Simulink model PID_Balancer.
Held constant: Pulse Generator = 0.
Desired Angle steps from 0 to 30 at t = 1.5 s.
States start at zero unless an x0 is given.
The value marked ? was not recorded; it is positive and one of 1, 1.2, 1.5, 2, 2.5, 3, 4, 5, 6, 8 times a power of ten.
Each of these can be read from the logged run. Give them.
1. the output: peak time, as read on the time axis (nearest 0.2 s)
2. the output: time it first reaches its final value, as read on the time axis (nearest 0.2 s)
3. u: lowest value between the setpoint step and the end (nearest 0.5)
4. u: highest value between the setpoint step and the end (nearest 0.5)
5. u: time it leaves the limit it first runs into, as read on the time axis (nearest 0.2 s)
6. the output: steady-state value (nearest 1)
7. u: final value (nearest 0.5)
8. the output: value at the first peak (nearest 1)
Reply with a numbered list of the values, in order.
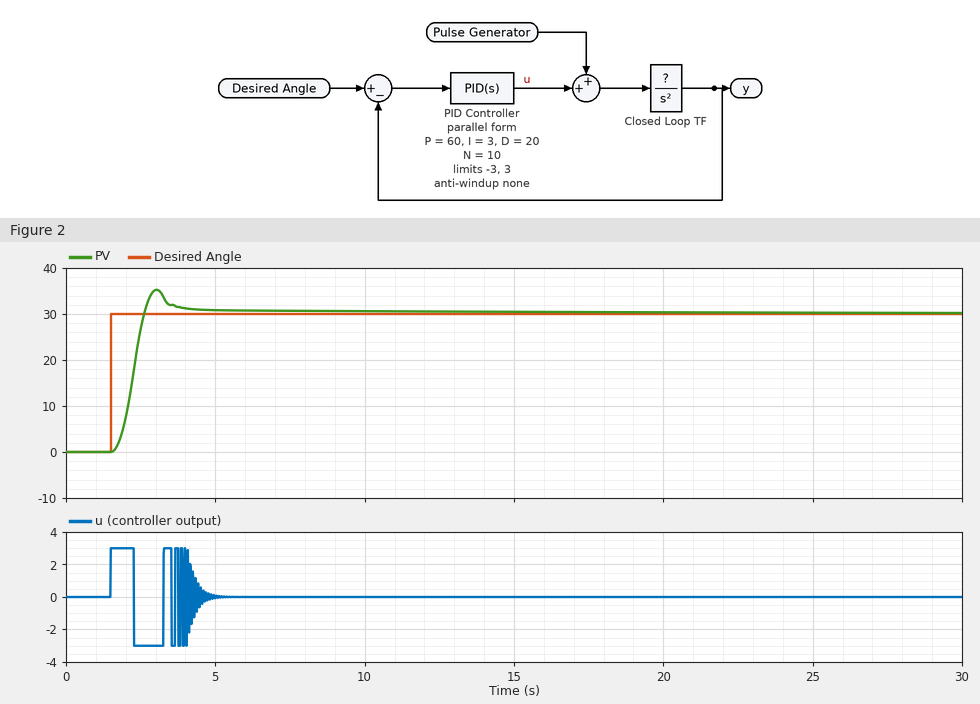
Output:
1. 3.0 s
2. 2.6 s
3. -3.0
4. 3.0
5. 2.2 s
6. 30
7. 0.0
8. 35
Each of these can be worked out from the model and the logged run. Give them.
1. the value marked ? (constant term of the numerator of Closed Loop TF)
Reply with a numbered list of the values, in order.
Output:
1. 20
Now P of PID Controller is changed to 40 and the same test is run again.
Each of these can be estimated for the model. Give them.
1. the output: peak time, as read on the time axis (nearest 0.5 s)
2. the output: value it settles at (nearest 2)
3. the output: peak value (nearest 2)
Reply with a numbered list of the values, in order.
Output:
1. 5.5 s
2. 30
3. 32
